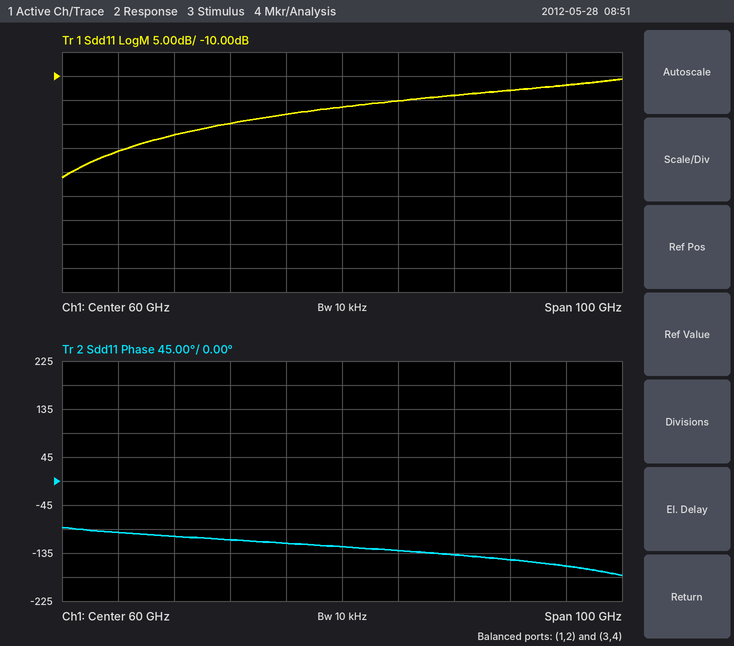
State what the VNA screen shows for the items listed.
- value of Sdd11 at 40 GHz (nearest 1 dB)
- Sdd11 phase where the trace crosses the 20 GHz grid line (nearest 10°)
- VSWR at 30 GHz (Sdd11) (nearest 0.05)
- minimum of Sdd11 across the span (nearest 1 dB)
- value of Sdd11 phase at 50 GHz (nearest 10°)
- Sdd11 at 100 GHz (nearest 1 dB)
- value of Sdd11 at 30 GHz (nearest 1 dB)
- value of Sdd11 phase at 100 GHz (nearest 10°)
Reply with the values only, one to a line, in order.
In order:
-20 dB
-100°
1.15
-31 dB
-120°
-12 dB
-22 dB
-160°
